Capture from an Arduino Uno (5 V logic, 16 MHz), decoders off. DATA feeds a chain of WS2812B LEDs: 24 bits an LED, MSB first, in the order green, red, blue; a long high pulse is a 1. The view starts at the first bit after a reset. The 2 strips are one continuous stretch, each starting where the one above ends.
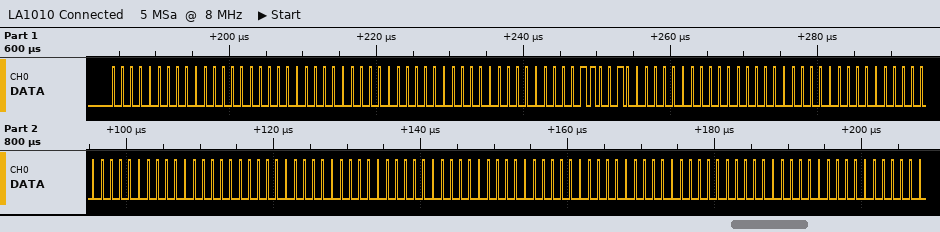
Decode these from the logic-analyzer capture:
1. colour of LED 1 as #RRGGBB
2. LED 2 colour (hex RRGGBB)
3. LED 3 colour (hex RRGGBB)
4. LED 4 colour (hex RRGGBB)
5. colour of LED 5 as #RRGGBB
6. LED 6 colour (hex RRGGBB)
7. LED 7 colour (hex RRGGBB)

#000000
#000000
#001900
#000000
#000000
#000000
#000000
